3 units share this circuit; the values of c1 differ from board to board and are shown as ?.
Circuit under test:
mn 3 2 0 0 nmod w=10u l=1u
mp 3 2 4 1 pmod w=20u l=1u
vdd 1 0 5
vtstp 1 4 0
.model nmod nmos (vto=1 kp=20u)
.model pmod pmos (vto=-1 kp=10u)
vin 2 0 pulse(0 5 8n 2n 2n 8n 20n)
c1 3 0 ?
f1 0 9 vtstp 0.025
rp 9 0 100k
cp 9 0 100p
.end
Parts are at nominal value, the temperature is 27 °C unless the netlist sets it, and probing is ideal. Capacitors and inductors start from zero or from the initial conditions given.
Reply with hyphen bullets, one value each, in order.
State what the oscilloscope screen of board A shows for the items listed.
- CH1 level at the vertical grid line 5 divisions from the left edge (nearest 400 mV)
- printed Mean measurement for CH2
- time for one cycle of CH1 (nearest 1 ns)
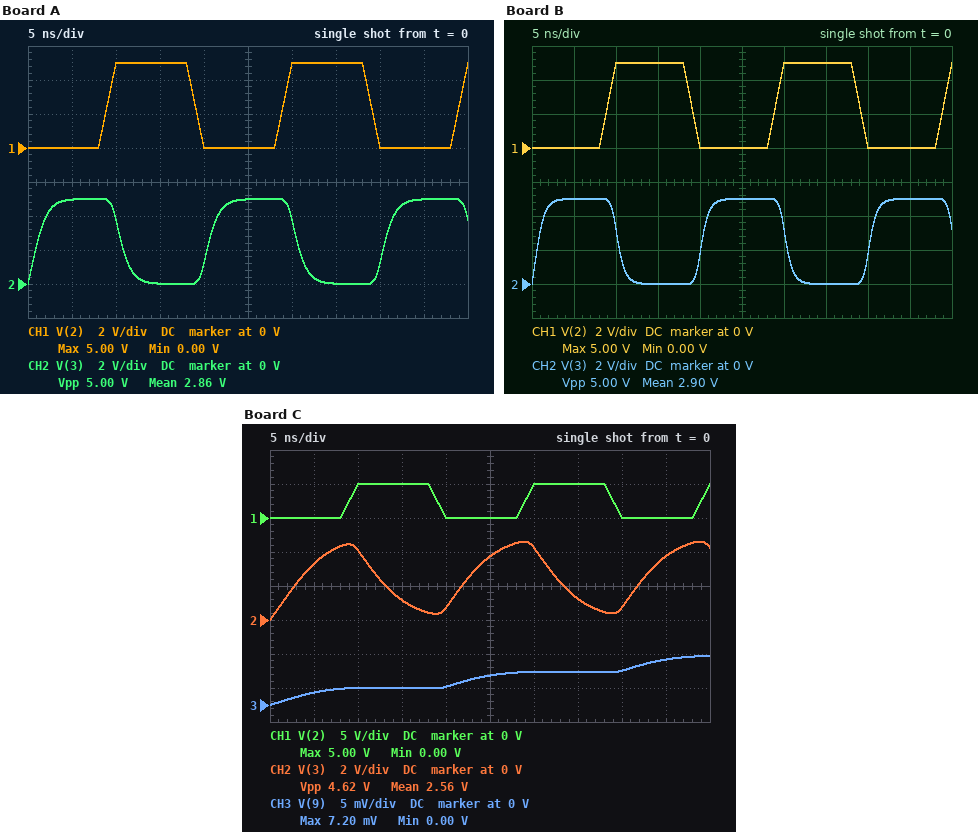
- 0 V
- 2.86 V
- 20 ns
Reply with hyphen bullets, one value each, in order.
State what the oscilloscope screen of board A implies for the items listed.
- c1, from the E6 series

- 680 fF
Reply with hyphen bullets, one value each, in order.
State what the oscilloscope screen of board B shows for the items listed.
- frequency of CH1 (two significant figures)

- 50 MHz
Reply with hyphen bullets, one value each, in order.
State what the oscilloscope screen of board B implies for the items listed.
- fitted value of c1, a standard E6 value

- 470 fF
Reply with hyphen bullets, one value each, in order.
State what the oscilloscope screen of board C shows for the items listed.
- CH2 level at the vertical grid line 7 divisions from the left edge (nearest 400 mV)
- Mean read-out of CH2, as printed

- 1.2 V
- 2.56 V
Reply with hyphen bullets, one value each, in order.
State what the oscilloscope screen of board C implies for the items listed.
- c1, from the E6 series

- 2.2 pF
